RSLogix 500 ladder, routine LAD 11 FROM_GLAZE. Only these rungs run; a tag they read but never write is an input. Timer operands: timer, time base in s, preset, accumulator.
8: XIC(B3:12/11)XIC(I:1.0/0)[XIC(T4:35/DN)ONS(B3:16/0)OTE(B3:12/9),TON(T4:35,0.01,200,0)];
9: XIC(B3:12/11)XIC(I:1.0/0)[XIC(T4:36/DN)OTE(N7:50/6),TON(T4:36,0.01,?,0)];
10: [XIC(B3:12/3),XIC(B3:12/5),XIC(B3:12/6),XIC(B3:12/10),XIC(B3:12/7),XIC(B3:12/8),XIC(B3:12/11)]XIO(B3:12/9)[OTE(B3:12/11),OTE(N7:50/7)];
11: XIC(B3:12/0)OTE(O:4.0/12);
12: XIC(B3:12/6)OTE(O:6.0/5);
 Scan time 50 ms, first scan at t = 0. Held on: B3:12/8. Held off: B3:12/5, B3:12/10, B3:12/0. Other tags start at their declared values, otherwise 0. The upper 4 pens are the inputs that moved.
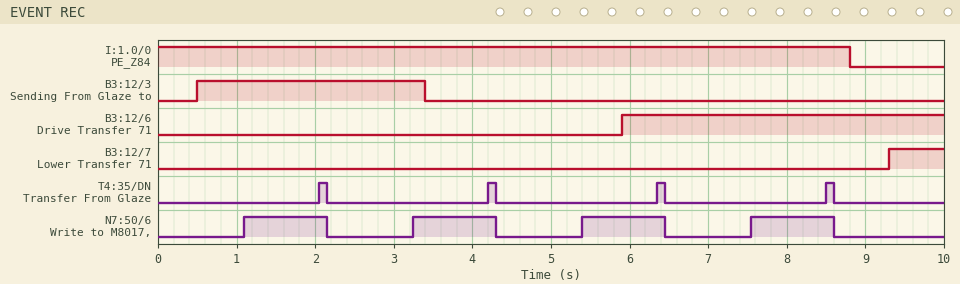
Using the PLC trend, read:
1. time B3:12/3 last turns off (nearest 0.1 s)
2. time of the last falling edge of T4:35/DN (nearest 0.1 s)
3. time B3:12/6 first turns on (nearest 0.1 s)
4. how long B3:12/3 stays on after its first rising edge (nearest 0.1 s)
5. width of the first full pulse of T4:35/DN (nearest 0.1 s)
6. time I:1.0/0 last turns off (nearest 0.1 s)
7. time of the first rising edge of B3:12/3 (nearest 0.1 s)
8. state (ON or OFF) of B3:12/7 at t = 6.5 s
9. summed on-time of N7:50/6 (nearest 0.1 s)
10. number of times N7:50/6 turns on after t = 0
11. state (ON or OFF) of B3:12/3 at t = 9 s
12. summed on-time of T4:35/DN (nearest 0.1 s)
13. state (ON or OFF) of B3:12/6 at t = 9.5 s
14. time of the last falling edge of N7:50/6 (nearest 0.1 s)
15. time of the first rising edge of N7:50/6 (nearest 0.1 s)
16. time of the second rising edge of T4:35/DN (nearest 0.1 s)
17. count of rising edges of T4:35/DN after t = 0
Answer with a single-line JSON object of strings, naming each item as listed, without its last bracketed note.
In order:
{"time B3:12/3 last turns off": "3.4 s", "time of the last falling edge of T4:35/DN": "8.6 s", "time B3:12/6 first turns on": "5.9 s", "how long B3:12/3 stays on after its first rising edge": "2.9 s", "width of the first full pulse of T4:35/DN": "0.1 s", "time I:1.0/0 last turns off": "8.8 s", "time of the first rising edge of B3:12/3": "0.5 s", "state (ON or OFF) of B3:12/7 at t = 6.5 s": "OFF", "summed on-time of N7:50/6": "4.2 s", "number of times N7:50/6 turns on after t = 0": "4", "state (ON or OFF) of B3:12/3 at t = 9 s": "OFF", "summed on-time of T4:35/DN": "0.4 s", "state (ON or OFF) of B3:12/6 at t = 9.5 s": "ON", "time of the last falling edge of N7:50/6": "8.6 s", "time of the first rising edge of N7:50/6": "1.1 s", "time of the second rising edge of T4:35/DN": "4.2 s", "count of rising edges of T4:35/DN after t = 0": "4"}
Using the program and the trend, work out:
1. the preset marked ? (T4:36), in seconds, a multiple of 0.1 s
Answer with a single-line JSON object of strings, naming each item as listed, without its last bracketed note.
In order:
{"the preset marked ? (T4:36), in seconds, a multiple of 0.1 s": "1.0 s"}
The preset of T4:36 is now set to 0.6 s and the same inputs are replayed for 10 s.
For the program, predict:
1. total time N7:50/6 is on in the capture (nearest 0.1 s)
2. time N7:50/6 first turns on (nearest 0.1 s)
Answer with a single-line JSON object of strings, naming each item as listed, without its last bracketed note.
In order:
{"total time N7:50/6 is on in the capture": "5.8 s", "time N7:50/6 first turns on": "0.7 s"}
